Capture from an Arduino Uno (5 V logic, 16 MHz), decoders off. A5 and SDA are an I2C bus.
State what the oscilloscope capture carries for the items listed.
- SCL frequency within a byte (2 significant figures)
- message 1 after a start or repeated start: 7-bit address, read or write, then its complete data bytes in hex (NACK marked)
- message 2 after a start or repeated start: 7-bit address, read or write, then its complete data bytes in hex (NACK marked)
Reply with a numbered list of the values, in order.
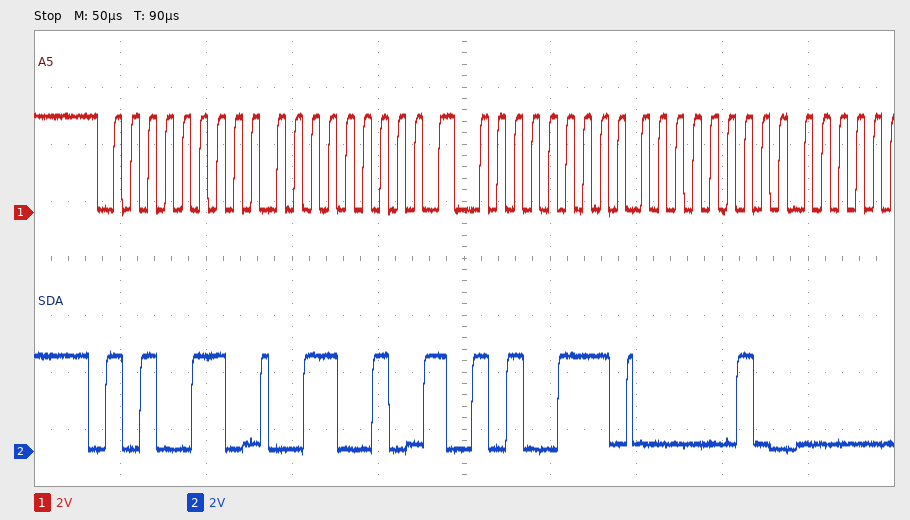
1. 100 kHz
2. 0x53 write: 32
3. 0x53 read: 02
